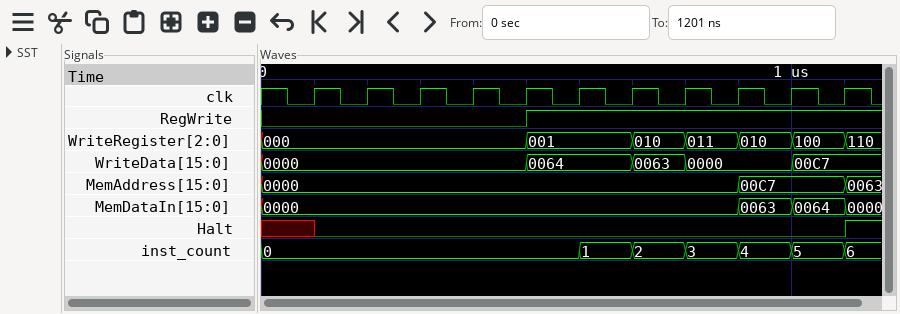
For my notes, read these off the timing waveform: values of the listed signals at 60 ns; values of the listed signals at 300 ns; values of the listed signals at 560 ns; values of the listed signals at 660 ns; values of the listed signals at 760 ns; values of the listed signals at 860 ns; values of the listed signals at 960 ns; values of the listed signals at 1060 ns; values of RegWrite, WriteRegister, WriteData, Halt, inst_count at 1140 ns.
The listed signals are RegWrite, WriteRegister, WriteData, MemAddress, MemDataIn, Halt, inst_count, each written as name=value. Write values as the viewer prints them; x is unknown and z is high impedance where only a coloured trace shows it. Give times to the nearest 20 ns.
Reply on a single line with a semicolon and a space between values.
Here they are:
RegWrite=0, WriteRegister=000, WriteData=0000, MemAddress=0000, MemDataIn=0000, Halt=x, inst_count=0; RegWrite=0, WriteRegister=000, WriteData=0000, MemAddress=0000, MemDataIn=0000, Halt=0, inst_count=0; RegWrite=1, WriteRegister=001, WriteData=0064, MemAddress=0000, MemDataIn=0000, Halt=0, inst_count=0; RegWrite=1, WriteRegister=001, WriteData=0064, MemAddress=0000, MemDataIn=0000, Halt=0, inst_count=1; RegWrite=1, WriteRegister=010, WriteData=0063, MemAddress=0000, MemDataIn=0000, Halt=0, inst_count=2; RegWrite=1, WriteRegister=011, WriteData=0000, MemAddress=0000, MemDataIn=0000, Halt=0, inst_count=3; RegWrite=1, WriteRegister=010, WriteData=0000, MemAddress=00C7, MemDataIn=0063, Halt=0, inst_count=4; RegWrite=1, WriteRegister=100, WriteData=00C7, MemAddress=00C7, MemDataIn=0064, Halt=0, inst_count=5; RegWrite=1, WriteRegister=110, WriteData=00C7, Halt=1, inst_count=6
